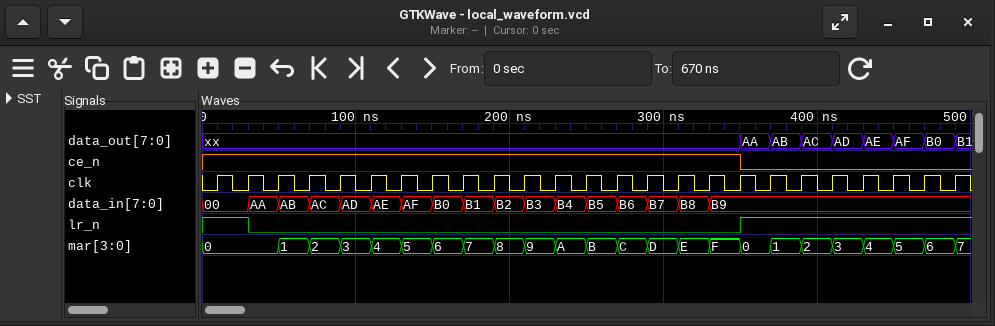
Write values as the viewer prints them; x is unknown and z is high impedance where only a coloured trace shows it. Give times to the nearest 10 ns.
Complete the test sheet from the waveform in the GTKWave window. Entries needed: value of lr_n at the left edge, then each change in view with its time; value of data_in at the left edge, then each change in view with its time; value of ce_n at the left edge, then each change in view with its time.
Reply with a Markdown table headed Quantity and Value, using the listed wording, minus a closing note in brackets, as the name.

| Quantity | Value |
|---|---|
| value of lr_n at the left edge, then each change in view with its time | 1, 0 at 30 ns, 1 at 350 ns |
| value of data_in at the left edge, then each change in view with its time | 00, AA at 30 ns, AB at 50 ns, AC at 70 ns, AD at 90 ns, AE at 110 ns, AF at 130 ns, B0 at 150 ns, B1 at 170 ns, B2 at 190 ns, B3 at 210 ns, B4 at 230 ns, B5 at 250 ns, B6 at 270 ns, B7 at 290 ns, B8 at 310 ns, B9 at 330 ns |
| value of ce_n at the left edge, then each change in view with its time | 1, 0 at 350 ns |
